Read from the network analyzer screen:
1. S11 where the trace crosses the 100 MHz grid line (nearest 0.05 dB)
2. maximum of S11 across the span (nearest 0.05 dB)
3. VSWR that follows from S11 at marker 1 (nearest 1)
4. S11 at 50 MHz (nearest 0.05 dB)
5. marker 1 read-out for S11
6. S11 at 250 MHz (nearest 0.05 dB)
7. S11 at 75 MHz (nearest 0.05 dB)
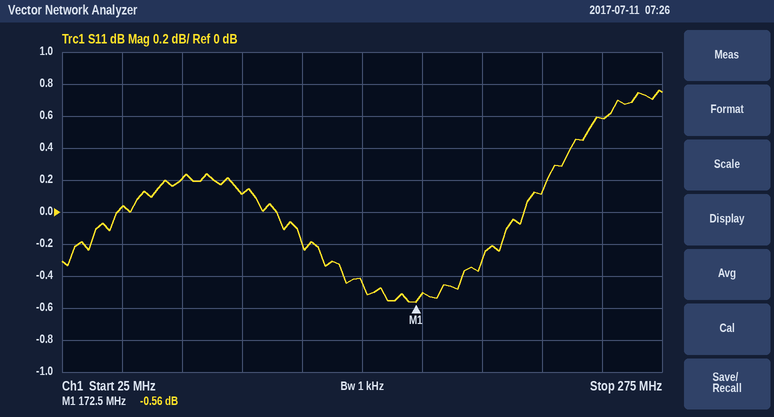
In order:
0.10 dB
0.75 dB
31
0.05 dB
-0.56 dB
0.60 dB
0.20 dB
